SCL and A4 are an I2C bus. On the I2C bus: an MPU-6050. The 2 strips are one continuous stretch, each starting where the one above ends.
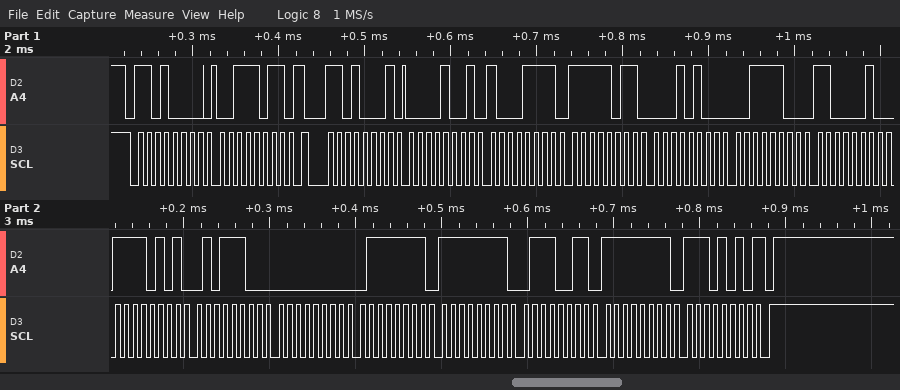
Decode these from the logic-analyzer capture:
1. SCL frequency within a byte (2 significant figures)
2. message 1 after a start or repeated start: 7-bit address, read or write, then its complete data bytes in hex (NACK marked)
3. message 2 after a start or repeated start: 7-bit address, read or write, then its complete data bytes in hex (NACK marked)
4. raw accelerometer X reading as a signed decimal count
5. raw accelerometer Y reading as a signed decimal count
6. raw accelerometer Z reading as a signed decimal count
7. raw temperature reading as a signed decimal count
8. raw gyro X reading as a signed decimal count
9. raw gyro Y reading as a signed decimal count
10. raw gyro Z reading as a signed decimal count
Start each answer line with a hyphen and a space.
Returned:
- 100 kHz
- 0x68 write: 3B
- 0x68 read: 09 8F FB 14 3C C2 F5 5C 00 7F FF 73 FF EA NACK
- 2447
- -1260
- 15554
- -2724
- 127
- -141
- -22
